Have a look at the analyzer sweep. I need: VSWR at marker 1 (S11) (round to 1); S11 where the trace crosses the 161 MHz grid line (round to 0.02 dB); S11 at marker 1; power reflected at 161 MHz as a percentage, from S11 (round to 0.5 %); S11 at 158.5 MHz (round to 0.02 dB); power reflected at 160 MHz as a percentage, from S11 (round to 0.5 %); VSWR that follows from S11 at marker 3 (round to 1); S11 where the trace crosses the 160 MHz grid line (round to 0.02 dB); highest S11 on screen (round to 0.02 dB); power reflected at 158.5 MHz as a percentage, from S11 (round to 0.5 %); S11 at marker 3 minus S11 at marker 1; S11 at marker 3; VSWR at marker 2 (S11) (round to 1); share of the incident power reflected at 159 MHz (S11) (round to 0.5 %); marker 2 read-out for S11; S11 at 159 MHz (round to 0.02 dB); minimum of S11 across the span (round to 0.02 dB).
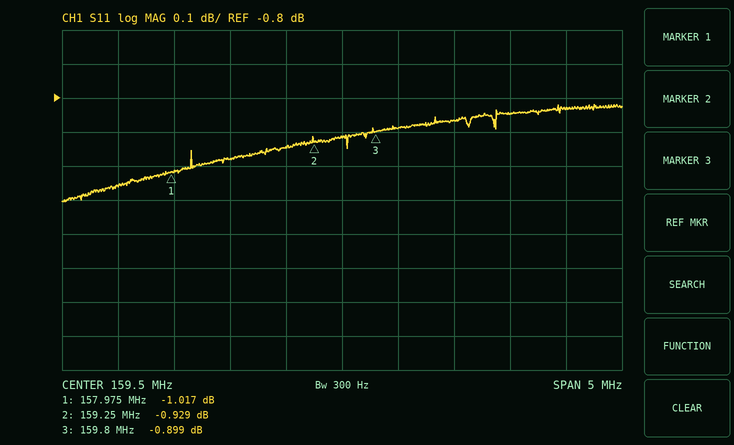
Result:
17
-0.84 dB
-1.017 dB
82.5 %
-0.98 dB
81.5 %
19
-0.88 dB
-0.82 dB
80.0 %
0.118 dB
-0.899 dB
19
80.5 %
-0.929 dB
-0.94 dB
-1.10 dB
